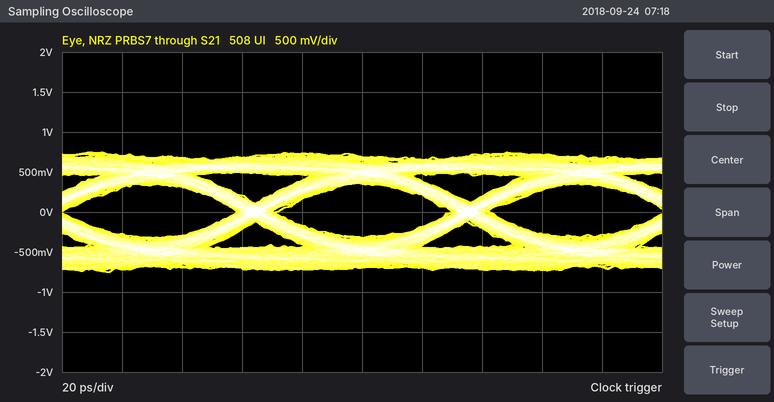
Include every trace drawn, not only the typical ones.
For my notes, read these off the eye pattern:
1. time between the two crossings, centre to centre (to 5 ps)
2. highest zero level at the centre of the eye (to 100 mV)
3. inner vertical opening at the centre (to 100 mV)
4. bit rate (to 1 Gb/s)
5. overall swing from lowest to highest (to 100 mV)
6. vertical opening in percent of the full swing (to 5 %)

70 ps
-300 mV
700 mV
14 Gb/s
1.5 V
45 %
